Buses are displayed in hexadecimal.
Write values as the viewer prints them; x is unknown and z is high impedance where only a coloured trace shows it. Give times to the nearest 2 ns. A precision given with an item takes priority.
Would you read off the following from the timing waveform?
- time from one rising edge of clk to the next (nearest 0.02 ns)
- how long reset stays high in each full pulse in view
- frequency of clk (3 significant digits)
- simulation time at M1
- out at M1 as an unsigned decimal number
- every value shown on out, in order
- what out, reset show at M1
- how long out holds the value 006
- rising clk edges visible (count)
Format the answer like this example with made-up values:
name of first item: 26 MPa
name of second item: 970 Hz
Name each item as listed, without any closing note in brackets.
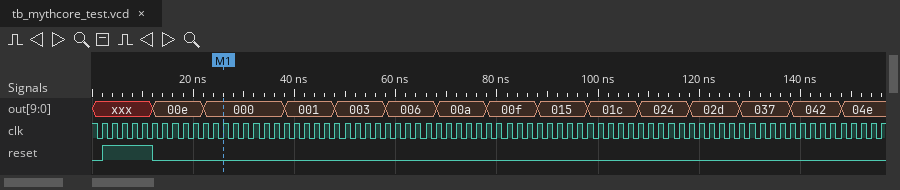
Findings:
time from one rising edge of clk to the next: 2 ns
how long reset stays high in each full pulse in view: 10 ns
frequency of clk: 500 MHz
simulation time at M1: 26 ns
out at M1 as an unsigned decimal number: 0
every value shown on out, in order: xxx, 00e, 000, 001, 003, 006, 00a, 00f, 015, 01c, 024, 02d, 037, 042, 04e
what out, reset show at M1: out=000, reset=0
how long out holds the value 006: 10 ns
rising clk edges visible: 78
